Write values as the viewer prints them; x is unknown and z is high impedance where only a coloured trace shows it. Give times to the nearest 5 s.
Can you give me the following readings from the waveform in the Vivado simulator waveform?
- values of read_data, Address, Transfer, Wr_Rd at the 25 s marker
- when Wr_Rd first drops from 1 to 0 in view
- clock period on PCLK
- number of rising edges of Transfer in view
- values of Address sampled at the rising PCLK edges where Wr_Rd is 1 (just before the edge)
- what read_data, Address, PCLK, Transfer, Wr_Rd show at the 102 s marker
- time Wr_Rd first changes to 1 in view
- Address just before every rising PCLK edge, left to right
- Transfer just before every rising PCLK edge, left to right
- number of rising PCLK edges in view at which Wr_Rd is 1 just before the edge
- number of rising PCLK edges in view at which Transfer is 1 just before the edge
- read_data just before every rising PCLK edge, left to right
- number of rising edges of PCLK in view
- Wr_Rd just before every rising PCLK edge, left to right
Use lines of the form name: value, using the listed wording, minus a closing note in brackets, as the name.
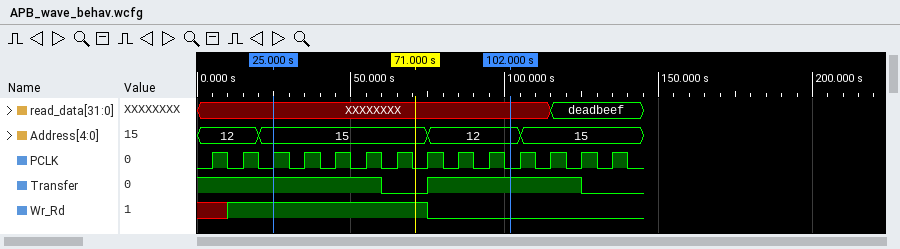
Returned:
values of read_data, Address, Transfer, Wr_Rd at the 25 s marker: read_data=XXXXXXXX, Address=15, Transfer=1, Wr_Rd=1
when Wr_Rd first drops from 1 to 0 in view: 75 s
clock period on PCLK: 10 s
number of rising edges of Transfer in view: 1
values of Address sampled at the rising PCLK edges where Wr_Rd is 1: 12, 15, 15, 15, 15, 15, 15
what read_data, Address, PCLK, Transfer, Wr_Rd show at the 102 s marker: read_data=XXXXXXXX, Address=12, PCLK=0, Transfer=1, Wr_Rd=0
time Wr_Rd first changes to 1 in view: 10 s
Address just before every rising PCLK edge, left to right: 12, 12, 15, 15, 15, 15, 15, 15, 12, 12, 12, 15, 15, 15
Transfer just before every rising PCLK edge, left to right: 1 1 1 1 1 1 0 0 1 1 1 1 1 0
number of rising PCLK edges in view at which Wr_Rd is 1 just before the edge: 7
number of rising PCLK edges in view at which Transfer is 1 just before the edge: 11
read_data just before every rising PCLK edge, left to right: XXXXXXXX, XXXXXXXX, XXXXXXXX, XXXXXXXX, XXXXXXXX, XXXXXXXX, XXXXXXXX, XXXXXXXX, XXXXXXXX, XXXXXXXX, XXXXXXXX, XXXXXXXX, deadbeef, deadbeef
number of rising edges of PCLK in view: 14
Wr_Rd just before every rising PCLK edge, left to right: x 1 1 1 1 1 1 1 0 0 0 0 0 0
